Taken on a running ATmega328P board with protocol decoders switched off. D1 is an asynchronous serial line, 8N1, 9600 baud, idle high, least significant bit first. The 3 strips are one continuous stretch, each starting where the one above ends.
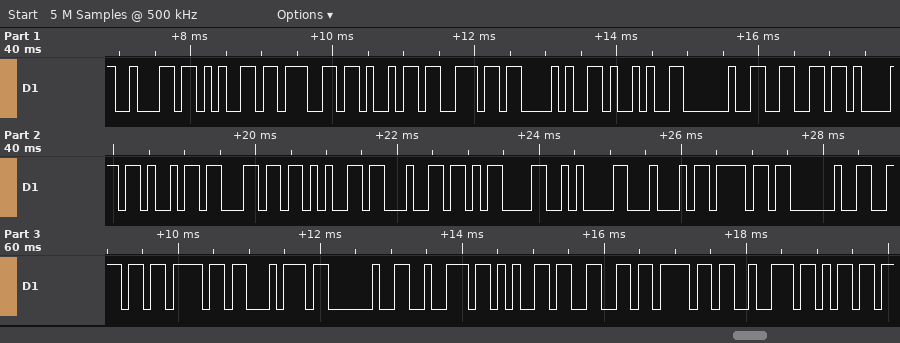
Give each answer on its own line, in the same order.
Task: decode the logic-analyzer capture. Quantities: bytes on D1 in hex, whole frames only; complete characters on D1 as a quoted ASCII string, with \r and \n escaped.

62 65 67 69 6E 28 29 20 66 61 69 6C 65 64 0D 0A 44 6F 20 6E 6F 74 20 72 65 66 6F 72 6D
"begin() failed\r\nDo not reform"
